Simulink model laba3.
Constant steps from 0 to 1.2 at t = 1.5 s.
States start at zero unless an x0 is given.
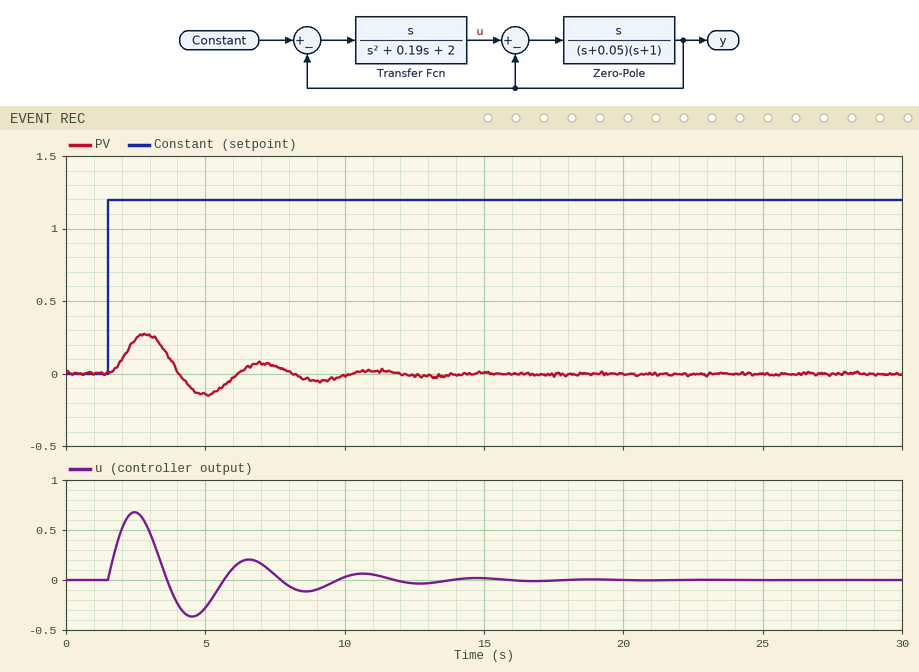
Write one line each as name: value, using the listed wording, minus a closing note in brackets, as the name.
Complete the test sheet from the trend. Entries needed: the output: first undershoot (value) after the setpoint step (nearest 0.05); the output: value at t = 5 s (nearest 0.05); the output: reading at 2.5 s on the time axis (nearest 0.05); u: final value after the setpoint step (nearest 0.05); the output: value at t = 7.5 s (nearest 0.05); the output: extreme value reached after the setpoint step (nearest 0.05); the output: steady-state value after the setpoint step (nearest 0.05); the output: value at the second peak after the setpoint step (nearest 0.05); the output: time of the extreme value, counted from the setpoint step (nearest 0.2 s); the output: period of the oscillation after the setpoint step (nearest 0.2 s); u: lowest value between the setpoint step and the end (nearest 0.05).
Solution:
the output: first undershoot (value) after the setpoint step: -0.15
the output: value at t = 5 s: -0.15
the output: reading at 2.5 s on the time axis: 0.25
u: final value after the setpoint step: 0.00
the output: value at t = 7.5 s: 0.05
the output: extreme value reached after the setpoint step: 0.25
the output: steady-state value after the setpoint step: 0.00
the output: value at the second peak after the setpoint step: 0.05
the output: time of the extreme value, counted from the setpoint step: 1.4 s
the output: period of the oscillation after the setpoint step: 4.2 s
u: lowest value between the setpoint step and the end: -0.35
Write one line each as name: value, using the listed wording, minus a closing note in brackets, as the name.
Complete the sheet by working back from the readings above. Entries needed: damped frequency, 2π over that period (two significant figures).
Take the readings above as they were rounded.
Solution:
damped frequency, 2π over that period: 1.5 rad/s
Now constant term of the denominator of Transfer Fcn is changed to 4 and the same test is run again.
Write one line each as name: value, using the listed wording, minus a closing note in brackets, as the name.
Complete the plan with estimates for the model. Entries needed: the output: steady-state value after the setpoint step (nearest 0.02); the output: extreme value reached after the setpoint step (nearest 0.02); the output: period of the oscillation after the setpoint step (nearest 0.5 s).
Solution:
the output: steady-state value after the setpoint step: 0.00
the output: extreme value reached after the setpoint step: 0.18
the output: period of the oscillation after the setpoint step: 3.0 s
